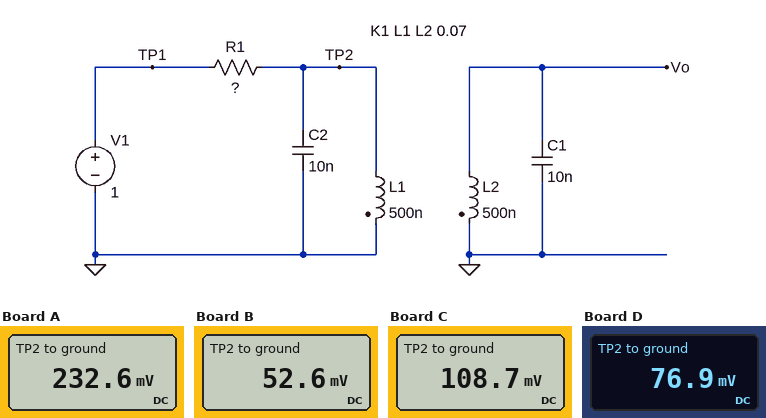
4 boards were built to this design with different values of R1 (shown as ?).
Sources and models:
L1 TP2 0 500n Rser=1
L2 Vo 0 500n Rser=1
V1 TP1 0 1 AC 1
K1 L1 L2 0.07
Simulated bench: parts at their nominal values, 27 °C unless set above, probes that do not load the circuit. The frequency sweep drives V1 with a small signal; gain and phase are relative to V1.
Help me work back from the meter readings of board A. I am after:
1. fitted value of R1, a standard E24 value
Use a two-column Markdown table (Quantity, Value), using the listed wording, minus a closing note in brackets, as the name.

| Quantity | Value |
|---|---|
| fitted value of R1, a standard E24 value | 3.3 Ω |
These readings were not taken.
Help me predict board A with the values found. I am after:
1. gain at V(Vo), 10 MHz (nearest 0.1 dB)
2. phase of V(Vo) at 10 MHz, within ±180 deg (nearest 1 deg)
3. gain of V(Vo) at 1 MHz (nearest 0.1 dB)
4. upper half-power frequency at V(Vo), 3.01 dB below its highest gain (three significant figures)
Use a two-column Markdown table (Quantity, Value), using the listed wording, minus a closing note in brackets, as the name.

| Quantity | Value |
|---|---|
| gain at V(Vo), 10 MHz | -55.4 dB |
| phase of V(Vo) at 10 MHz, within ±180 deg | 121 deg |
| gain of V(Vo) at 1 MHz | -25.2 dB |
| upper half-power frequency at V(Vo), 3.01 dB below its highest gain | 2.40 MHz |
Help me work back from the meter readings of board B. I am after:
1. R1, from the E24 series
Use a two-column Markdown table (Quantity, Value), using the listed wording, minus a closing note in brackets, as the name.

| Quantity | Value |
|---|---|
| R1, from the E24 series | 18 Ω |
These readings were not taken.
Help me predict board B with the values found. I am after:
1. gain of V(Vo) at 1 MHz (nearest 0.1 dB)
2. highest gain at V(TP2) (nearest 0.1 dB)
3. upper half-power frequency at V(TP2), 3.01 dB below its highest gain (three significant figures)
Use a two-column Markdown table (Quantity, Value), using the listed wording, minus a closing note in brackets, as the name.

| Quantity | Value |
|---|---|
| gain of V(Vo) at 1 MHz | -35.4 dB |
| highest gain at V(TP2) | -3.0 dB |
| upper half-power frequency at V(TP2), 3.01 dB below its highest gain | 3.06 MHz |
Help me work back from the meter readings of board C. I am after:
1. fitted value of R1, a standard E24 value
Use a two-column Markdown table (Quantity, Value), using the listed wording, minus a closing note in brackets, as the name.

| Quantity | Value |
|---|---|
| fitted value of R1, a standard E24 value | 8.2 Ω |
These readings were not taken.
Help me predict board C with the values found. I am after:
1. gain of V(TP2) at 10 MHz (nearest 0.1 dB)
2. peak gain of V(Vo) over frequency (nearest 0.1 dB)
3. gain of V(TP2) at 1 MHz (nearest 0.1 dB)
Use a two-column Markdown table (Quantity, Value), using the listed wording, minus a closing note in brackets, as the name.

| Quantity | Value |
|---|---|
| gain of V(TP2) at 10 MHz | -14.0 dB |
| peak gain of V(Vo) over frequency | -7.8 dB |
| gain of V(TP2) at 1 MHz | -8.1 dB |
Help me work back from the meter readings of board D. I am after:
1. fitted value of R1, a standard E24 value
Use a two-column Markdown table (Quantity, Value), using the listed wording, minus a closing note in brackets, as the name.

| Quantity | Value |
|---|---|
| fitted value of R1, a standard E24 value | 12 Ω |
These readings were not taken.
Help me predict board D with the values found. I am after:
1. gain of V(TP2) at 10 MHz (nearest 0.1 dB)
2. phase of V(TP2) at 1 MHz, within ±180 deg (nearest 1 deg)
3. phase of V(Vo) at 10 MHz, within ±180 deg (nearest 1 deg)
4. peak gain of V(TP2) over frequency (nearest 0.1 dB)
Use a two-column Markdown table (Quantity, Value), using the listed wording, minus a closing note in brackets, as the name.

| Quantity | Value |
|---|---|
| gain of V(TP2) at 10 MHz | -17.2 dB |
| phase of V(TP2) at 1 MHz, within ±180 deg | 52 deg |
| phase of V(Vo) at 10 MHz, within ±180 deg | 102 deg |
| peak gain of V(TP2) over frequency | -2.0 dB |
